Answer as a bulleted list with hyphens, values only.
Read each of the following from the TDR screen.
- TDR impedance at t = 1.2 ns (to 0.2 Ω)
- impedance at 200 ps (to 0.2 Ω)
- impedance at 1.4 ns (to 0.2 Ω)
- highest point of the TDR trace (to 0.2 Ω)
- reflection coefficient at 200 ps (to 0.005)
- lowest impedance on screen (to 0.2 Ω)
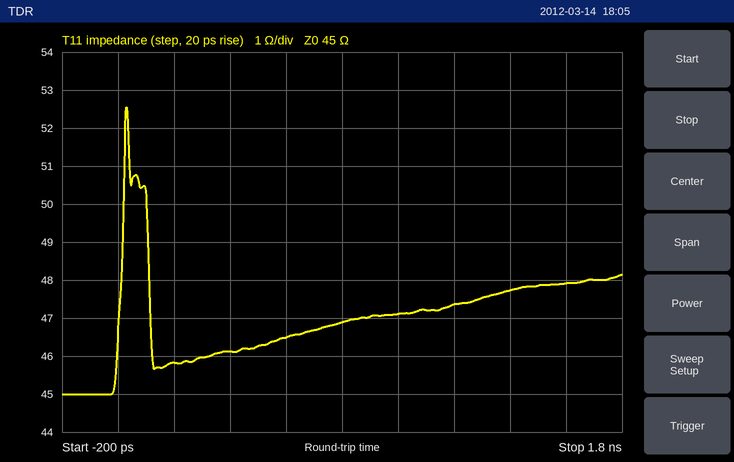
- 47.4 Ω
- 45.8 Ω
- 47.8 Ω
- 52.6 Ω
- +0.010
- 45.0 Ω
